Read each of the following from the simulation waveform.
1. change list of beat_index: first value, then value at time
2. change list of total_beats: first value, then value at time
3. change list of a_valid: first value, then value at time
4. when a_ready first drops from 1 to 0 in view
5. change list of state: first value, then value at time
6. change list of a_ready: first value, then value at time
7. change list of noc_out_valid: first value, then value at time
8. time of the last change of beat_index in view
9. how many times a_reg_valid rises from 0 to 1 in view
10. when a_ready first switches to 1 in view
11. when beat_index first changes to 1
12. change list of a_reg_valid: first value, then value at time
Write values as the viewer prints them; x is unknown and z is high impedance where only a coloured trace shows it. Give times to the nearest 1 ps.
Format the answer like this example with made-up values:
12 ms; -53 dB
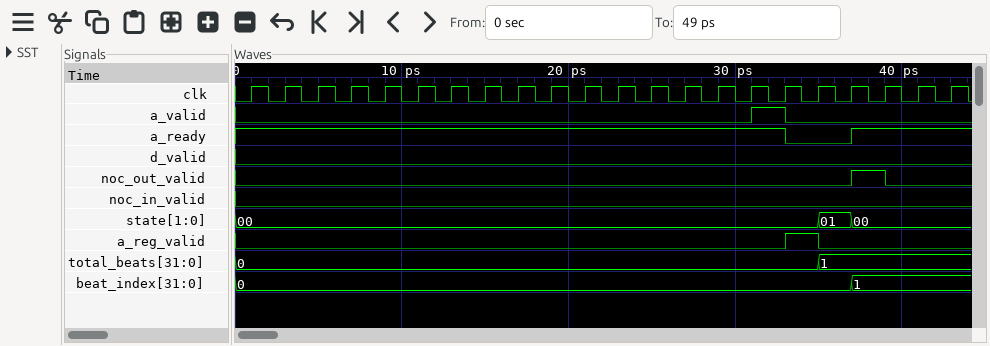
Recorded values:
0, 1 at 37 ps; 0, 1 at 35 ps; 0, 1 at 31 ps, 0 at 33 ps; 33 ps; 00, 01 at 35 ps, 00 at 37 ps; 1, 0 at 33 ps, 1 at 37 ps; 0, 1 at 37 ps, 0 at 39 ps; 37 ps; 1; 37 ps; 37 ps; 0, 1 at 33 ps, 0 at 35 ps
